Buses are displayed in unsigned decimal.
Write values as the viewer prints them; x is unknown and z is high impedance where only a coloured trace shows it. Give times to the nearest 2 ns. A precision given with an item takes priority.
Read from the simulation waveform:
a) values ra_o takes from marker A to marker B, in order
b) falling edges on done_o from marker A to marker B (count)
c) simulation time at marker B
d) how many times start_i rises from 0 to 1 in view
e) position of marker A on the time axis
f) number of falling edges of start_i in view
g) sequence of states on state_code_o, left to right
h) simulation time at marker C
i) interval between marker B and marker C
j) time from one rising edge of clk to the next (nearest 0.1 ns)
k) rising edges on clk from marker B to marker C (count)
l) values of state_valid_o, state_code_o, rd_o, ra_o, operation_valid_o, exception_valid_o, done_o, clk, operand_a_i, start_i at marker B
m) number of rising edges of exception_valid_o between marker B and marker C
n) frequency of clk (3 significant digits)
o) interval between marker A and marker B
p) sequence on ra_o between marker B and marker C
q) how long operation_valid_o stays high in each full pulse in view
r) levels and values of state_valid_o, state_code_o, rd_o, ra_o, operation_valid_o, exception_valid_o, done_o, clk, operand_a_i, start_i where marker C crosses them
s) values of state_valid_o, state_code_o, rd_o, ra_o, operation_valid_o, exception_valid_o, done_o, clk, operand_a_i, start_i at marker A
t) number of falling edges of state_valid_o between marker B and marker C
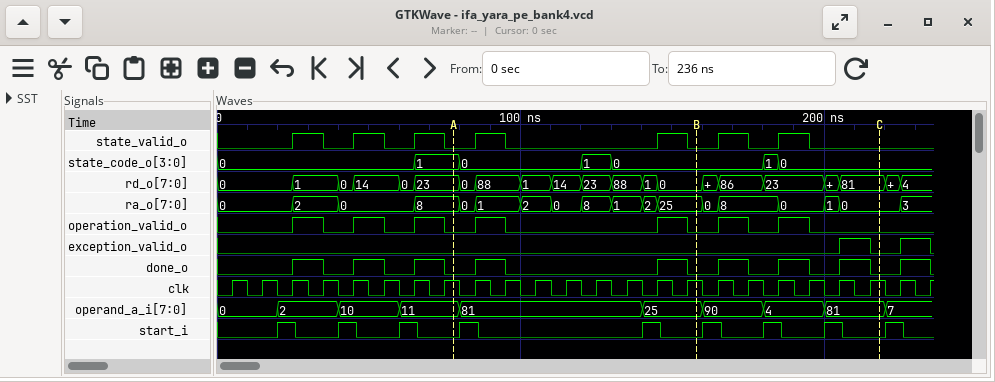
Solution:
8, 0, 1, 2, 0, 8, 1, 2, 25
2
158 ns
9
78 ns
9
0, 1, 0, 1, 0, 1, 0
218 ns
60 ns
10 ns
6
state_valid_o=0, state_code_o=0, rd_o=0, ra_o=25, operation_valid_o=0, exception_valid_o=0, done_o=0, clk=1, operand_a_i=25, start_i=0
1
100 MHz
80 ns
25, 0, 8, 0, 1, 0
10 ns, 10 ns, 10 ns, 10 ns, 10 ns, 10 ns, 10 ns
state_valid_o=0, state_code_o=0, rd_o=81, ra_o=0, operation_valid_o=0, exception_valid_o=0, done_o=0, clk=1, operand_a_i=81, start_i=0
state_valid_o=0, state_code_o=1, rd_o=23, ra_o=8, operation_valid_o=0, exception_valid_o=0, done_o=0, clk=1, operand_a_i=11, start_i=0
2
